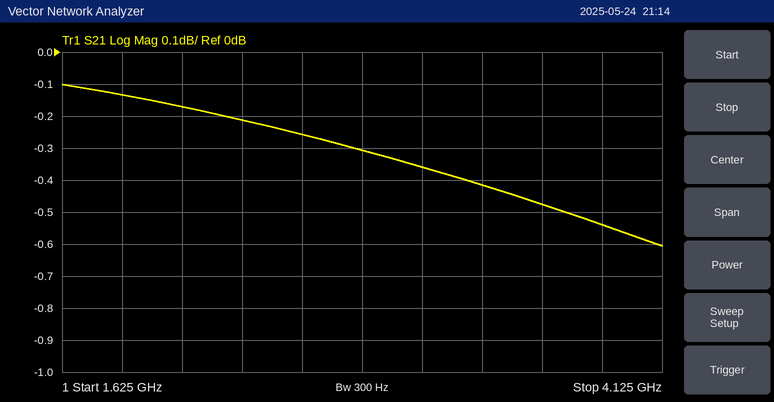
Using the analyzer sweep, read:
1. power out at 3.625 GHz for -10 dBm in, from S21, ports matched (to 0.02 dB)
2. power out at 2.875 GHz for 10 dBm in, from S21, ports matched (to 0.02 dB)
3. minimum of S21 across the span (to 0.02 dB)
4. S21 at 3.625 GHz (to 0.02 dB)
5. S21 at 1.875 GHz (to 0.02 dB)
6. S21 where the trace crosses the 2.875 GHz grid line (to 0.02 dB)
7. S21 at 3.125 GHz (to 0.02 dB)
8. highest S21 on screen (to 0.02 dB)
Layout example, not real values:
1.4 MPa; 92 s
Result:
-10.48 dBm; 9.70 dBm; -0.60 dB; -0.48 dB; -0.14 dB; -0.30 dB; -0.36 dB; -0.10 dB
